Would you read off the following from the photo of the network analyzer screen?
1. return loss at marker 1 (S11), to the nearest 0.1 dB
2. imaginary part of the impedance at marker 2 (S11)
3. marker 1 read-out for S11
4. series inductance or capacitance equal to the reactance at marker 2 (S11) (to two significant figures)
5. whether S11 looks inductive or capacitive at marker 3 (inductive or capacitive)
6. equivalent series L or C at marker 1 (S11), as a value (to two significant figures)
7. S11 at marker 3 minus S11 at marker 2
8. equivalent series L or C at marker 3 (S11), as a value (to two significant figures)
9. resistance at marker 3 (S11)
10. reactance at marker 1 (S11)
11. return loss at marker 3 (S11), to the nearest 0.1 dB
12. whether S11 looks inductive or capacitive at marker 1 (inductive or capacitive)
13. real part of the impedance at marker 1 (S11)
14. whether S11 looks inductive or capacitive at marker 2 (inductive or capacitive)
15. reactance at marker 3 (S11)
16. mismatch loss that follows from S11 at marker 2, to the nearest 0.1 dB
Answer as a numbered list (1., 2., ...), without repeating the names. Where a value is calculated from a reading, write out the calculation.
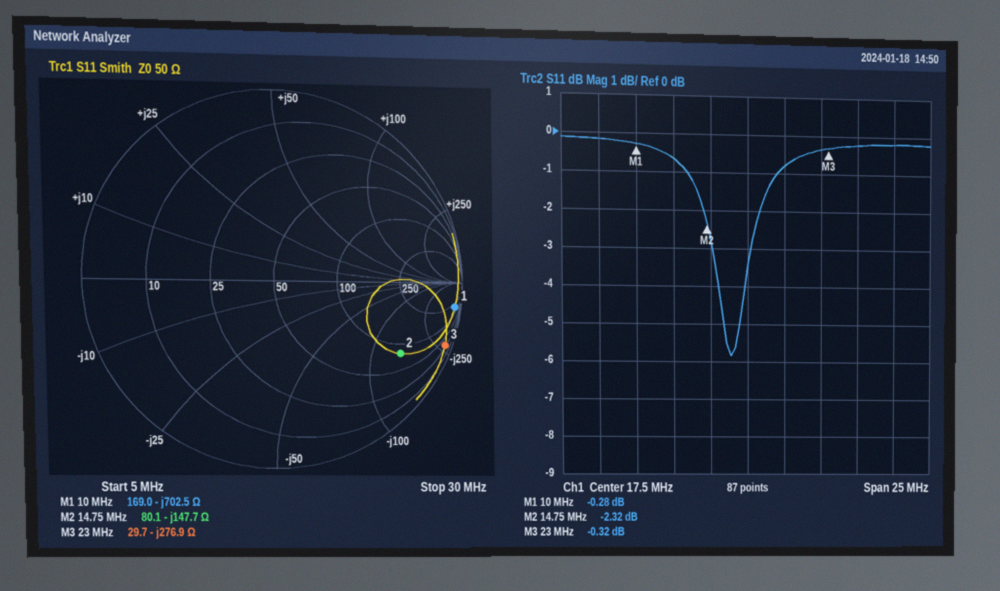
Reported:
1. 0.3 dB
2. -147.7 Ω
3. -0.28 dB
4. C = 1/(2π × 14.75 MHz × 147.7 Ω) ≈ 73 pF
5. capacitive
6. C = 1/(2π × 10 MHz × 702.5 Ω) ≈ 23 pF
7. -0.32 − (-2.32) = 2.00 dB
8. C = 1/(2π × 23 MHz × 276.9 Ω) ≈ 25 pF
9. 29.7 Ω
10. -702.5 Ω
11. 0.3 dB
12. capacitive
13. 169.0 Ω
14. capacitive
15. -276.9 Ω
16. −10 log10(1 − 10^(-2.32/10)) ≈ 3.8 dB
